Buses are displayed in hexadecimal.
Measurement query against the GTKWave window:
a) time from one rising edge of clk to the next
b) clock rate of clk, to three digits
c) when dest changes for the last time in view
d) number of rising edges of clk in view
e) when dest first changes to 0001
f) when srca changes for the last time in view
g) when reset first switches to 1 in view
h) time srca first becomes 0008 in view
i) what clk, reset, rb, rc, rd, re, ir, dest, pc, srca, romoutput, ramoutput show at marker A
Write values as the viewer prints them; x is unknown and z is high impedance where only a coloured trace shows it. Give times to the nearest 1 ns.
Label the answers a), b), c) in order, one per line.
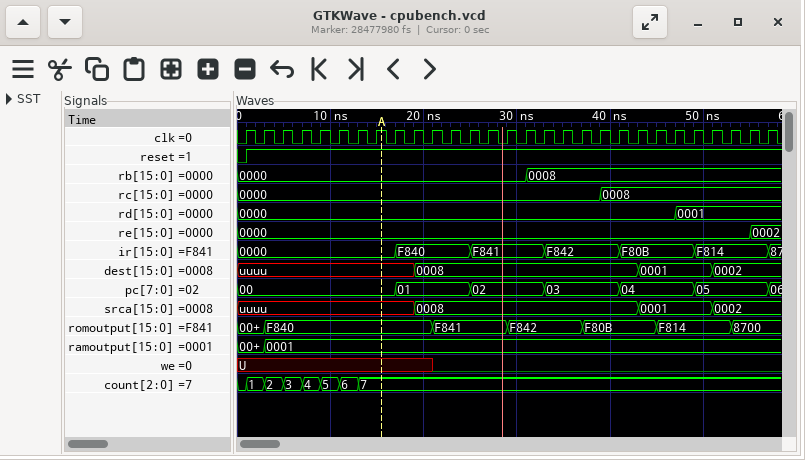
a) 2 ns
b) 500 MHz
c) 51 ns
d) 29
e) 43 ns
f) 51 ns
g) 1 ns
h) 19 ns
i) clk=1, reset=1, rb=0000, rc=0000, rd=0000, re=0000, ir=0000, dest=uuuu, pc=00, srca=uuuu, romoutput=F840, ramoutput=0001
